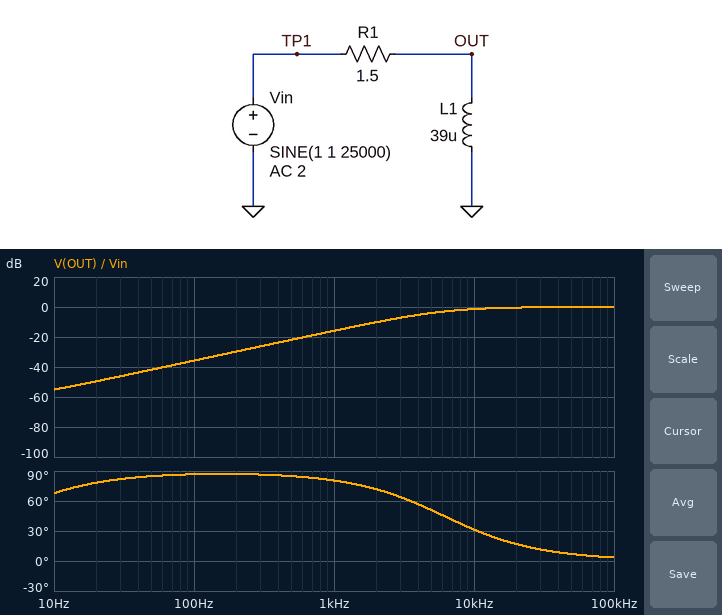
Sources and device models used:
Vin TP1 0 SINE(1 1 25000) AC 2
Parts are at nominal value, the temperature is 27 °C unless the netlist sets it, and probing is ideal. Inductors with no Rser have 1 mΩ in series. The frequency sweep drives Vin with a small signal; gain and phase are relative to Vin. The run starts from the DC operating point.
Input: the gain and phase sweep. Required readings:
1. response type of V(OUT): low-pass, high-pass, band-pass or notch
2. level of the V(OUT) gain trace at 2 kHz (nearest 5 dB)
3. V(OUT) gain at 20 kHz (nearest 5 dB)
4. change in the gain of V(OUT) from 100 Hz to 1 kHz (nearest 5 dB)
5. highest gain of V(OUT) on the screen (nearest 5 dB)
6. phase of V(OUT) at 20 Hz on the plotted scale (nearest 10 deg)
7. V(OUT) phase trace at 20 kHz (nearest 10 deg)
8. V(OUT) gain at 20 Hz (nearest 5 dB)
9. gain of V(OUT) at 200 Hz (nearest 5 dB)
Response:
high-pass
-10 dB
0 dB
20 dB
0 dB
80 deg
20 deg
-50 dB
-30 dB
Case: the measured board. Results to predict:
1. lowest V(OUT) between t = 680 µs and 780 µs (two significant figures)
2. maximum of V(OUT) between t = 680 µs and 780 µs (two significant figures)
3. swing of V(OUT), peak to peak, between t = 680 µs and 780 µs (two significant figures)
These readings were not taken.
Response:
-970 mV
970 mV
1.9 V
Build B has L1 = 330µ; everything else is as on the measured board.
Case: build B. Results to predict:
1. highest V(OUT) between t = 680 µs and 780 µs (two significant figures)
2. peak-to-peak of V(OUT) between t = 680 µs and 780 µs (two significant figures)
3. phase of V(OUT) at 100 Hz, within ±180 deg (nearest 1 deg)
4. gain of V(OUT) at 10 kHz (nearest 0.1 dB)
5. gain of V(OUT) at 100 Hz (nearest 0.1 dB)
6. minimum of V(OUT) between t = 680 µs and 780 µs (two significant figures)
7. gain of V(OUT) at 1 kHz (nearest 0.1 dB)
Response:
1.0 V
2.0 V
82 deg
0 dB
-17.3 dB
-1.0 V
-1.8 dB
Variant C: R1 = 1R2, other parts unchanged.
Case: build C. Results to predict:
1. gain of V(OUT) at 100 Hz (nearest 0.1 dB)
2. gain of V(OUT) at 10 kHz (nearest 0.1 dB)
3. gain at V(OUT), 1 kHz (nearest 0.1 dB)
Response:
-33.8 dB
-0.9 dB
-14.0 dB
